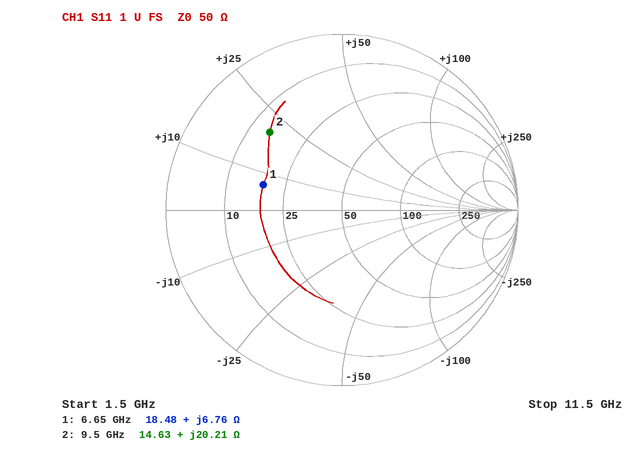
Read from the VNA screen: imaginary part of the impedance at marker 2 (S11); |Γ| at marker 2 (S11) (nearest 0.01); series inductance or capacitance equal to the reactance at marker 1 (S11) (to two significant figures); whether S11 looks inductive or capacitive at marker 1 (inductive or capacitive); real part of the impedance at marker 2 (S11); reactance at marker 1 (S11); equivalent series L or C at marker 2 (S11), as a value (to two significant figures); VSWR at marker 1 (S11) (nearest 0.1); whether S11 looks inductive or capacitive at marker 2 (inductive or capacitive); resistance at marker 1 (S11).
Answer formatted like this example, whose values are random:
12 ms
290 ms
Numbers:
+20.21 Ω
0.60
160 pH
inductive
14.63 Ω
+6.76 Ω
340 pH
2.8
inductive
18.48 Ω
